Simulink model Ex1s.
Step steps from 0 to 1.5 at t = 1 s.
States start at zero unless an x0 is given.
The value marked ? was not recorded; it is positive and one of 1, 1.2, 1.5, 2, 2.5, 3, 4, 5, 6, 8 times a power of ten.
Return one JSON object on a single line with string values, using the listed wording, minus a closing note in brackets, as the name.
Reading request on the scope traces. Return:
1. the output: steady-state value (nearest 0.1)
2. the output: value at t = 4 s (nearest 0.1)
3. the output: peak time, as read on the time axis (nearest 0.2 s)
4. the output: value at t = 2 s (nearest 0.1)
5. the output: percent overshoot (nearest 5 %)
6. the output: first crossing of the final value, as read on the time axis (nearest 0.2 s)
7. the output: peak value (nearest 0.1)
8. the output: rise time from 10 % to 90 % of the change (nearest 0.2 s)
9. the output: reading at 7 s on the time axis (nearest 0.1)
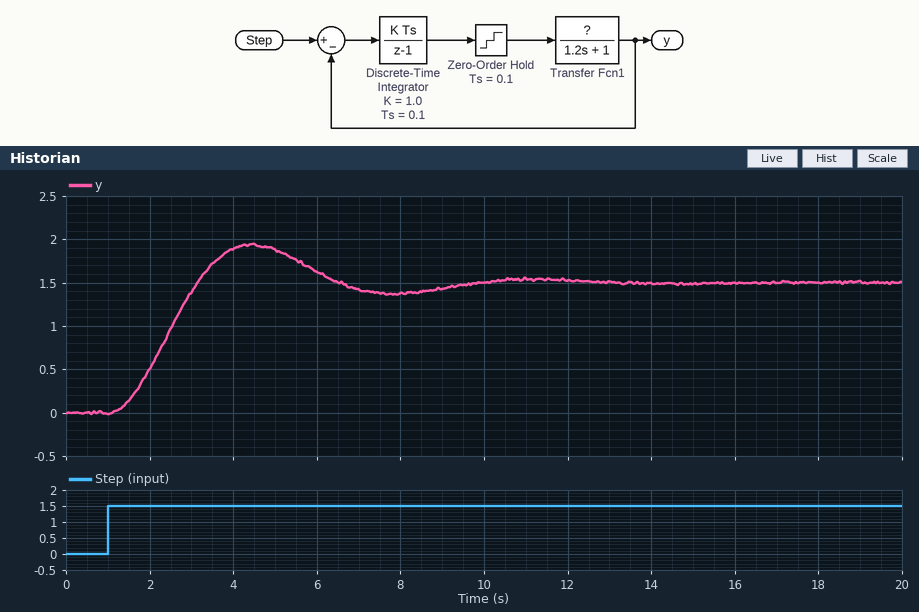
{"the output: steady-state value": "1.5", "the output: value at t = 4 s": "1.9", "the output: peak time, as read on the time axis": "4.4 s", "the output: value at t = 2 s": "0.5", "the output: percent overshoot": "30 %", "the output: first crossing of the final value, as read on the time axis": "3.2 s", "the output: peak value": "1.9", "the output: rise time from 10 % to 90 % of the change": "1.4 s", "the output: reading at 7 s on the time axis": "1.4"}
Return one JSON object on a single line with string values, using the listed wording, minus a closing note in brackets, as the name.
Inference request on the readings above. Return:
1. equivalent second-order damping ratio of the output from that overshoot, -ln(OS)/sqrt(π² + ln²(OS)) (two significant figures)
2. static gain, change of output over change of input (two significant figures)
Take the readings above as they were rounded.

{"equivalent second-order damping ratio of the output from that overshoot, -ln(OS)/sqrt(π² + ln²(OS))": "0.36", "static gain, change of output over change of input": "1.0"}
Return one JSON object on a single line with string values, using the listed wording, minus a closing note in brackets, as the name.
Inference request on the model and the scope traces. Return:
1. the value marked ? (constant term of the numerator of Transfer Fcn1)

{"the value marked ?": "1.2"}
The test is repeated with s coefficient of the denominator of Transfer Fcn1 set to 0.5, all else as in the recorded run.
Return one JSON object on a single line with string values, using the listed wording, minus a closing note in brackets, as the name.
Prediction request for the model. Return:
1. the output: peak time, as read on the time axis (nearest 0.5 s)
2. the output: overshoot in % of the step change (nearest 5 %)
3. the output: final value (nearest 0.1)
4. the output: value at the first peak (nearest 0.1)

{"the output: peak time, as read on the time axis": "3.5 s", "the output: overshoot in % of the step change": "10 %", "the output: final value": "1.5", "the output: value at the first peak": "1.7"}
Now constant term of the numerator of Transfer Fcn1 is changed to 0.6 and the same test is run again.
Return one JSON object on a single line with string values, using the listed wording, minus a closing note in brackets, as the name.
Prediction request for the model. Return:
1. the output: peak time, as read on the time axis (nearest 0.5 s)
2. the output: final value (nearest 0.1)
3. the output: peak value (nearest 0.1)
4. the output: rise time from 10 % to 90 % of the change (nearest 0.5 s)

{"the output: peak time, as read on the time axis": "6.5 s", "the output: final value": "1.5", "the output: peak value": "1.7", "the output: rise time from 10 % to 90 % of the change": "2.5 s"}
